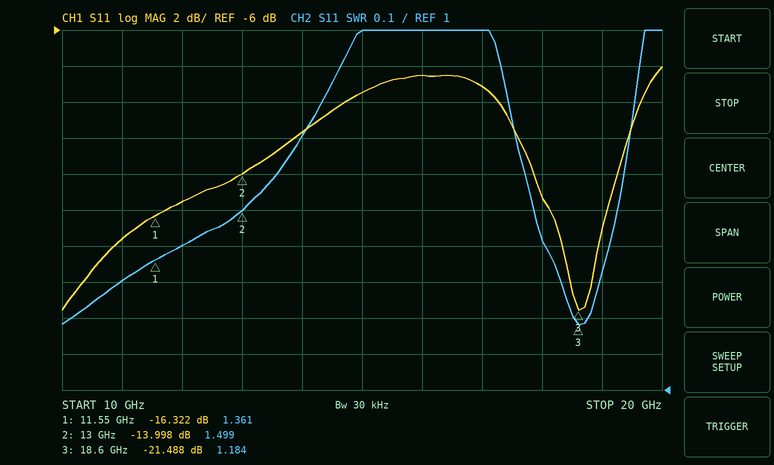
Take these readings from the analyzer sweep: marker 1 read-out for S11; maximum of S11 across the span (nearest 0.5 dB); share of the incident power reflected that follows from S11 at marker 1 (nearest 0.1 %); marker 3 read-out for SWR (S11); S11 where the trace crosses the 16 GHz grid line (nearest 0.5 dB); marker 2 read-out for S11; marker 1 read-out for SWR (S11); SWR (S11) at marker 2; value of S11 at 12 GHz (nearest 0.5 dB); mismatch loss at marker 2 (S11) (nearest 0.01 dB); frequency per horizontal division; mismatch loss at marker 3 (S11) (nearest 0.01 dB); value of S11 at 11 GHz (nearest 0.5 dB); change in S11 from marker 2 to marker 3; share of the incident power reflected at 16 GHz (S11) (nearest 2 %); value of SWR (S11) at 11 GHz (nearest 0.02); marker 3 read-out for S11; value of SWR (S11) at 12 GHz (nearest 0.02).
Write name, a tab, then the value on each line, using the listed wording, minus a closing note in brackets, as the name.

marker 1 read-out for S11	-16.322 dB
maximum of S11 across the span	-8.0 dB
share of the incident power reflected that follows from S11 at marker 1	2.3 %
marker 3 read-out for SWR	1.184
S11 where the trace crosses the 16 GHz grid line	-8.5 dB
marker 2 read-out for S11	-13.998 dB
marker 1 read-out for SWR	1.361
SWR (S11) at marker 2	1.499
value of S11 at 12 GHz	-15.5 dB
mismatch loss at marker 2 (S11)	0.18 dB
frequency per horizontal division	1 GHz
mismatch loss at marker 3 (S11)	0.03 dB
value of S11 at 11 GHz	-17.5 dB
change in S11 from marker 2 to marker 3	-7.490 dB
share of the incident power reflected at 16 GHz (S11)	14 %
value of SWR (S11) at 11 GHz	1.30
marker 3 read-out for S11	-21.488 dB
value of SWR (S11) at 12 GHz	1.40
